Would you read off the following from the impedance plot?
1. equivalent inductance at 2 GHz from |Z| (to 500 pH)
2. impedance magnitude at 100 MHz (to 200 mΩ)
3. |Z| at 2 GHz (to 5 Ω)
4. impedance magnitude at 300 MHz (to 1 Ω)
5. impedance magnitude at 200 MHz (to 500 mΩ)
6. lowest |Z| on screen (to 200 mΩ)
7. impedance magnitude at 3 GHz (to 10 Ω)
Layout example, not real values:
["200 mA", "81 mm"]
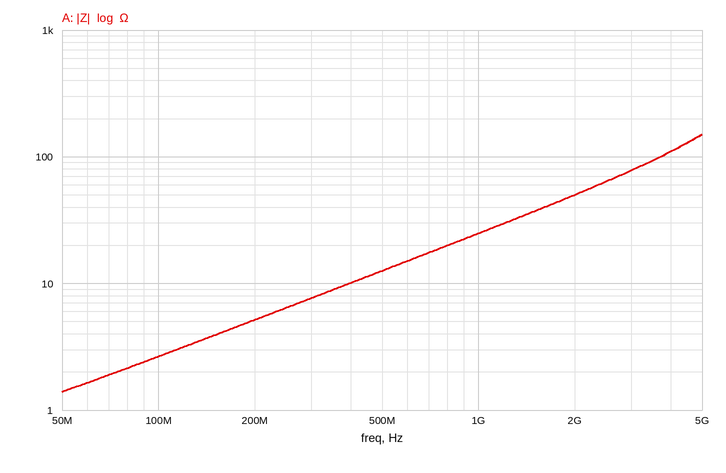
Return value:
["4.0 nH", "2.6 Ω", "50 Ω", "8 Ω", "5.0 Ω", "1.4 Ω", "80 Ω"]
